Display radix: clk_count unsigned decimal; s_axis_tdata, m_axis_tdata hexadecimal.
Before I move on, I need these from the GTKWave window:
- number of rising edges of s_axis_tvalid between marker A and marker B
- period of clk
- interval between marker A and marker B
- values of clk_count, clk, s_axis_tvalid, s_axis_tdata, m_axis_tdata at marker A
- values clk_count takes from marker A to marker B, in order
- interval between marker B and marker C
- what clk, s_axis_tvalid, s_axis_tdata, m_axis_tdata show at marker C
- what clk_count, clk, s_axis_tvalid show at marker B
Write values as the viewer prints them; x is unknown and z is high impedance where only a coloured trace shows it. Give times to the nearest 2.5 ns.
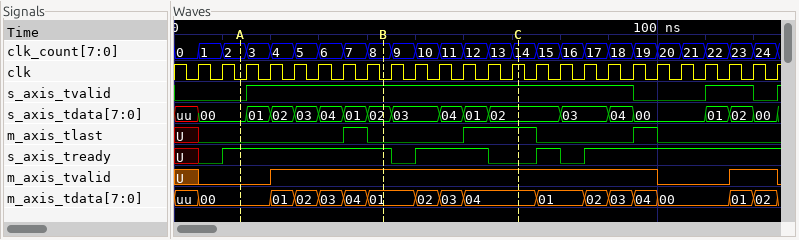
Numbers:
1
5 ns
30 ns
clk_count=2, clk=0, s_axis_tvalid=0, s_axis_tdata=00, m_axis_tdata=00
2, 3, 4, 5, 6, 7, 8
27.5 ns
clk=1, s_axis_tvalid=1, s_axis_tdata=02, m_axis_tdata=04
clk_count=8, clk=0, s_axis_tvalid=1
